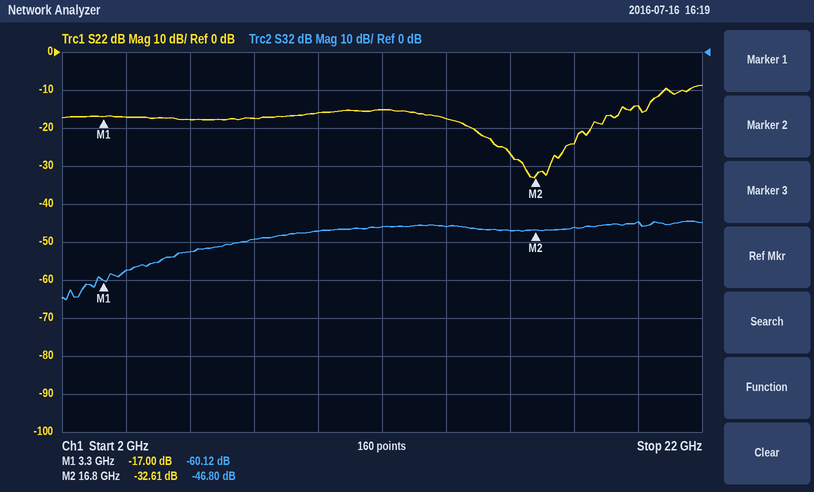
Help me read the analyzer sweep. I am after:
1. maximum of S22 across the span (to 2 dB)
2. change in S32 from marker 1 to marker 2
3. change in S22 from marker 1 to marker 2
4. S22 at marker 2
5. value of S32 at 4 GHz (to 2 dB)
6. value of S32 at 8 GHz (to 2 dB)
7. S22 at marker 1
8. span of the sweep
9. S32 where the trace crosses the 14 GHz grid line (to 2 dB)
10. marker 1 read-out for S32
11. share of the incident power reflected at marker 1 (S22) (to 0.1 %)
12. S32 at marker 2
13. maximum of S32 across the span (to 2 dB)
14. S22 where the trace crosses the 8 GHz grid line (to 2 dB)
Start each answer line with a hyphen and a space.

- -8 dB
- 13.32 dB
- -15.61 dB
- -32.61 dB
- -58 dB
- -50 dB
- -17.00 dB
- 20 GHz
- -46 dB
- -60.12 dB
- 2.0 %
- -46.80 dB
- -44 dB
- -18 dB
